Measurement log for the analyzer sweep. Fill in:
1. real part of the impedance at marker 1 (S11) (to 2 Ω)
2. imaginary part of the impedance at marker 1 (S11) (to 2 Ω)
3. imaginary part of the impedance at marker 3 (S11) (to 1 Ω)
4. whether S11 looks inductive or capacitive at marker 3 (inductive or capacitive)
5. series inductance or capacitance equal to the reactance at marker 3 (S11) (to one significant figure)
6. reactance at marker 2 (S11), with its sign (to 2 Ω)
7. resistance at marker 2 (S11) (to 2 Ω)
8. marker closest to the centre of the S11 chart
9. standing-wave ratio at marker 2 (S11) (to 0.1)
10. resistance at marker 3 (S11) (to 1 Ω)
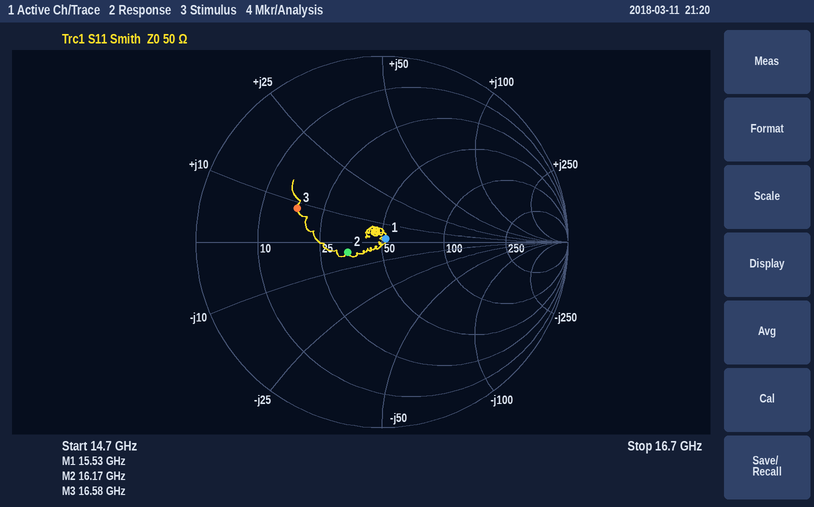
52 Ω
+2 Ω
+8 Ω
inductive
80 pH
-4 Ω
34 Ω
marker 1
1.5
18 Ω
